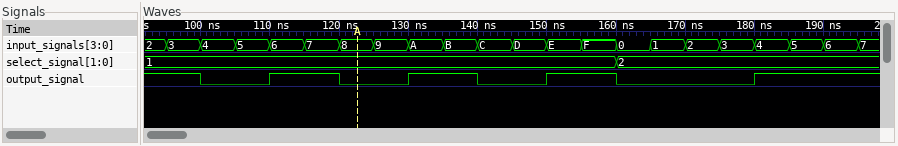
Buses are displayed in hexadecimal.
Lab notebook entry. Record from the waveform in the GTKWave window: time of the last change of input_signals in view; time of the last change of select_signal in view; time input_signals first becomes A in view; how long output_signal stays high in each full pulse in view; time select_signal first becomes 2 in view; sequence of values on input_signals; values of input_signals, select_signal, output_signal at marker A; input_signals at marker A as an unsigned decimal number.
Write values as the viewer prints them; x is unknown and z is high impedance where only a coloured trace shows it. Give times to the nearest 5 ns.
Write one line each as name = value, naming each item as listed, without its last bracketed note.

time of the last change of input_signals in view = 195 ns
time of the last change of select_signal in view = 160 ns
time input_signals first becomes A in view = 130 ns
how long output_signal stays high in each full pulse in view = 10 ns, 10 ns, 10 ns
time select_signal first becomes 2 in view = 160 ns
sequence of values on input_signals = 2, 3, 4, 5, 6, 7, 8, 9, A, B, C, D, E, F, 0, 1, 2, 3, 4, 5, 6, 7
values of input_signals, select_signal, output_signal at marker A = input_signals=8, select_signal=1, output_signal=0
input_signals at marker A as an unsigned decimal number = 8
